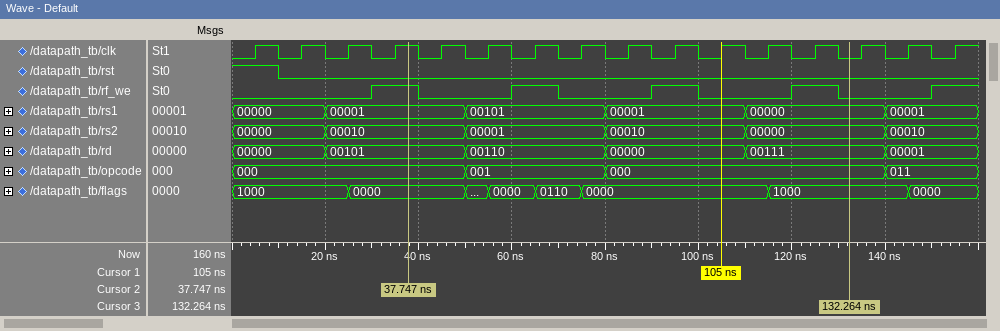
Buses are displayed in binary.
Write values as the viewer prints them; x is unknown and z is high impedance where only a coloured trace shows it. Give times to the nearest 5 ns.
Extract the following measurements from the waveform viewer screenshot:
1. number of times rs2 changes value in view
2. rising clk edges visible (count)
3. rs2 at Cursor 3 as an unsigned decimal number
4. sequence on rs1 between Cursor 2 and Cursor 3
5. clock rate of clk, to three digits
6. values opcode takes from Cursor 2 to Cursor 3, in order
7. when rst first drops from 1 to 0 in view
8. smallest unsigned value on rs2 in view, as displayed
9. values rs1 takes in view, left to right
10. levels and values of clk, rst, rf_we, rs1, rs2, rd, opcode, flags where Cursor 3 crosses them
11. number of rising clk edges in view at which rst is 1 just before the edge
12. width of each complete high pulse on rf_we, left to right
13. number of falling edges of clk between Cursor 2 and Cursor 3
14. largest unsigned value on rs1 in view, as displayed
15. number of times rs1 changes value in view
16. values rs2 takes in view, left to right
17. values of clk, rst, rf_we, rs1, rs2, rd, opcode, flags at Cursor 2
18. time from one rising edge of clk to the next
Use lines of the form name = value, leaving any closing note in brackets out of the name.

number of times rs2 changes value in view = 5
rising clk edges visible = 16
rs2 at Cursor 3 as an unsigned decimal number = 0
sequence on rs1 between Cursor 2 and Cursor 3 = 00001, 00101, 00001, 00000
clock rate of clk, to three digits = 100 MHz
values opcode takes from Cursor 2 to Cursor 3, in order = 000, 001, 000
when rst first drops from 1 to 0 in view = 10 ns
smallest unsigned value on rs2 in view, as displayed = 00000
values rs1 takes in view, left to right = 00000, 00001, 00101, 00001, 00000, 00001
levels and values of clk, rst, rf_we, rs1, rs2, rd, opcode, flags where Cursor 3 crosses them = clk=0, rst=0, rf_we=0, rs1=00000, rs2=00000, rd=00111, opcode=000, flags=1000
number of rising clk edges in view at which rst is 1 just before the edge = 1
width of each complete high pulse on rf_we, left to right = 10 ns, 10 ns, 10 ns, 10 ns
number of falling edges of clk between Cursor 2 and Cursor 3 = 10
largest unsigned value on rs1 in view, as displayed = 00101
number of times rs1 changes value in view = 5
values rs2 takes in view, left to right = 00000, 00010, 00001, 00010, 00000, 00010
values of clk, rst, rf_we, rs1, rs2, rd, opcode, flags at Cursor 2 = clk=1, rst=0, rf_we=1, rs1=00001, rs2=00010, rd=00101, opcode=000, flags=0000
time from one rising edge of clk to the next = 10 ns
